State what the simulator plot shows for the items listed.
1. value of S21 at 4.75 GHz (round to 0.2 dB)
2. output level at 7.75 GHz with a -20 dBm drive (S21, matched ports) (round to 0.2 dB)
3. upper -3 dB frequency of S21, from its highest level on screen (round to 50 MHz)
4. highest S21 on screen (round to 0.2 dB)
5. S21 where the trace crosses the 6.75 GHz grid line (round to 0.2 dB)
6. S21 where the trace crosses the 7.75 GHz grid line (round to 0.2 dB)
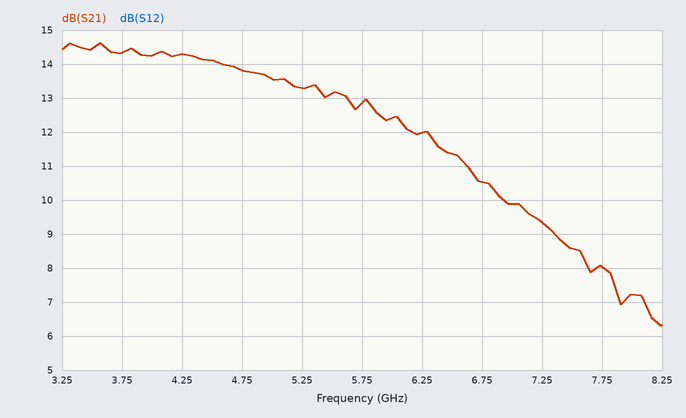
13.8 dB
-12.0 dBm
6.35 GHz
14.6 dB
10.6 dB
8.0 dB
